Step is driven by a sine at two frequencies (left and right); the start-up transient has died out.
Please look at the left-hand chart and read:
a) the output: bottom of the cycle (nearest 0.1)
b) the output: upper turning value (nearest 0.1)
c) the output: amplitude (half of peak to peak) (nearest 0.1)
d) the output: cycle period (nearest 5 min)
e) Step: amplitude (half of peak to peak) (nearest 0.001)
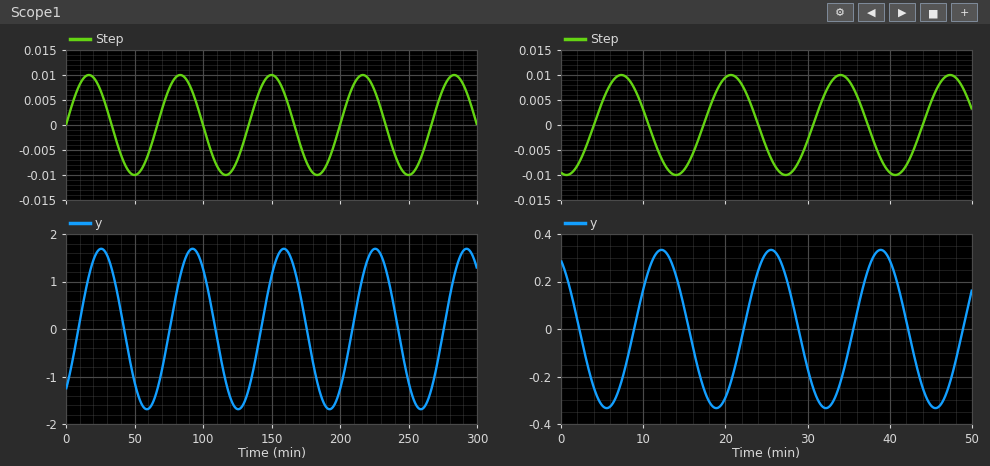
-1.7
1.7
1.7
65 min
0.010
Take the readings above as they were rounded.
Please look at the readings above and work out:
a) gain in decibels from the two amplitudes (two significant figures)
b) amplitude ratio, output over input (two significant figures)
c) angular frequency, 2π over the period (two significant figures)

45 dB
170
0.097 rad/min
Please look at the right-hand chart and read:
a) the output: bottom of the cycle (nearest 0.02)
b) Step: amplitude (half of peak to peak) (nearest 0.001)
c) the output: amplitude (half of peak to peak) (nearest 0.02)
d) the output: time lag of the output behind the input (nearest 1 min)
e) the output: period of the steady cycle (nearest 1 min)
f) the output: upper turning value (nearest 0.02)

-0.34
0.010
0.34
5 min
13 min
0.34
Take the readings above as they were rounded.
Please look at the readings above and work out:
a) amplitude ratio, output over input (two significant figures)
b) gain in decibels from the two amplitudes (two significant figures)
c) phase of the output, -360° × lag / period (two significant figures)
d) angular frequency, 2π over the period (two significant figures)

34
31 dB
-140°
0.48 rad/min
